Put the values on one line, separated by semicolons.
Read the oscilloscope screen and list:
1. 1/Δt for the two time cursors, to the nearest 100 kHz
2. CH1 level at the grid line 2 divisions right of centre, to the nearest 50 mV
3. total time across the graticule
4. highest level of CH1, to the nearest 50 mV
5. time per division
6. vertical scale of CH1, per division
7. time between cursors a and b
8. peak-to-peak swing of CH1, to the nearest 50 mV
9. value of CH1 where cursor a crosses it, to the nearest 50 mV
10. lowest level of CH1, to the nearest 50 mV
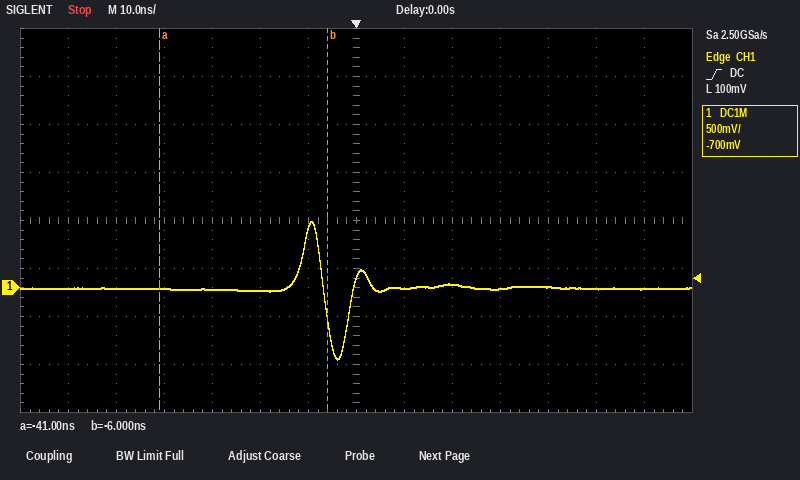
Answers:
28.6 MHz; 50 mV; 140 ns; 700 mV; 10 ns; 500 mV; 35 ns; 1.45 V; 0 mV; -750 mV
